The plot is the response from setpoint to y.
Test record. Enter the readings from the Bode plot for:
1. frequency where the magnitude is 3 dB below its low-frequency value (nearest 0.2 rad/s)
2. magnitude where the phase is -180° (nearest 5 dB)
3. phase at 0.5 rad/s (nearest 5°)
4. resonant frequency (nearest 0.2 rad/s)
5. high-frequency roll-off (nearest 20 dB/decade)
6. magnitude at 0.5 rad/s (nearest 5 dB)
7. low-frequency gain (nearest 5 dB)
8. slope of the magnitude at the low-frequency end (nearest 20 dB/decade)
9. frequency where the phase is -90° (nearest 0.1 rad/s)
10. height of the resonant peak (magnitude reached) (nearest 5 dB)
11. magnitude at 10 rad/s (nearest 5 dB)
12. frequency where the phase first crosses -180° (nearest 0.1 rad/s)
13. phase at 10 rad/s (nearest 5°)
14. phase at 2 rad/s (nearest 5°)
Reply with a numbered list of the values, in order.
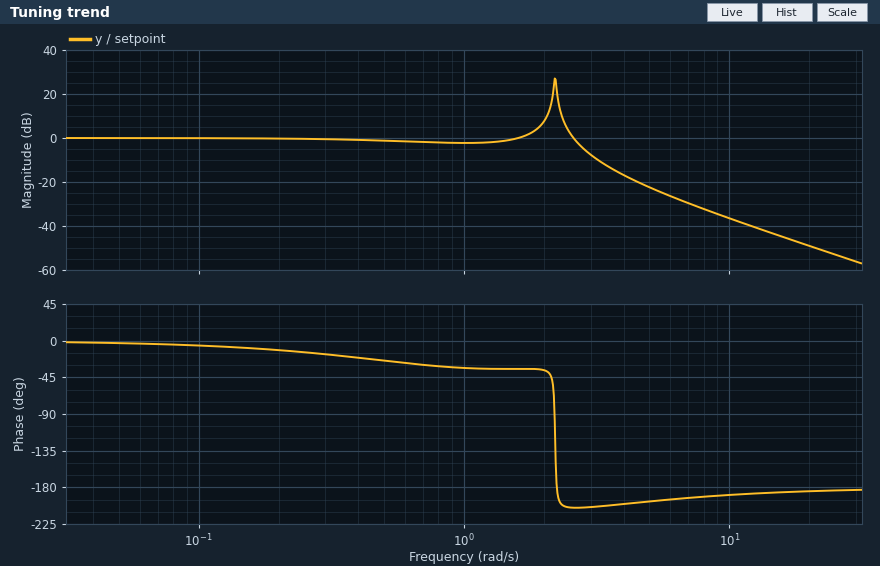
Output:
1. 2.8 rad/s
2. 20 dB
3. -25°
4. 2.2 rad/s
5. -40 dB/decade
6. 0 dB
7. 0 dB
8. 0 dB/decade
9. 2.2 rad/s
10. 25 dB
11. -35 dB
12. 2.2 rad/s
13. -190°
14. -35°
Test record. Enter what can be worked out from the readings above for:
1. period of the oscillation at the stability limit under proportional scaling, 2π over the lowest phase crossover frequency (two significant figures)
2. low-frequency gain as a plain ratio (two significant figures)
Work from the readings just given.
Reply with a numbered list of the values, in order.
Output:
1. 2.9 s
2. 1.0
